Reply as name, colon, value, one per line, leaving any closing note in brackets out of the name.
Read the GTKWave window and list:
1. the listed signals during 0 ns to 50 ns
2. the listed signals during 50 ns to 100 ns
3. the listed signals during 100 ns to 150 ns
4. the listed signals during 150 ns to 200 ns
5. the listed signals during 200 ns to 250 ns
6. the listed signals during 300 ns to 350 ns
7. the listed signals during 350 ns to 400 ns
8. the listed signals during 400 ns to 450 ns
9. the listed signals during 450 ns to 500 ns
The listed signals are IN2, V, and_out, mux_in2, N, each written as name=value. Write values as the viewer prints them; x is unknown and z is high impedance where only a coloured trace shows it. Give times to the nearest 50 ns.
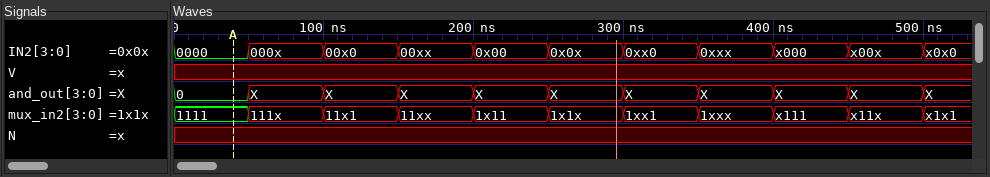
the listed signals during 0 ns to 50 ns: IN2=0000, V=x, and_out=0, mux_in2=1111, N=x
the listed signals during 50 ns to 100 ns: IN2=000x, V=x, and_out=X, mux_in2=111x, N=x
the listed signals during 100 ns to 150 ns: IN2=00x0, V=x, and_out=X, mux_in2=11x1, N=x
the listed signals during 150 ns to 200 ns: IN2=00xx, V=x, and_out=X, mux_in2=11xx, N=x
the listed signals during 200 ns to 250 ns: IN2=0x00, V=x, and_out=X, mux_in2=1x11, N=x
the listed signals during 300 ns to 350 ns: IN2=0xx0, V=x, and_out=X, mux_in2=1xx1, N=x
the listed signals during 350 ns to 400 ns: IN2=0xxx, V=x, and_out=X, mux_in2=1xxx, N=x
the listed signals during 400 ns to 450 ns: IN2=x000, V=x, and_out=X, mux_in2=x111, N=x
the listed signals during 450 ns to 500 ns: IN2=x00x, V=x, and_out=X, mux_in2=x11x, N=x
